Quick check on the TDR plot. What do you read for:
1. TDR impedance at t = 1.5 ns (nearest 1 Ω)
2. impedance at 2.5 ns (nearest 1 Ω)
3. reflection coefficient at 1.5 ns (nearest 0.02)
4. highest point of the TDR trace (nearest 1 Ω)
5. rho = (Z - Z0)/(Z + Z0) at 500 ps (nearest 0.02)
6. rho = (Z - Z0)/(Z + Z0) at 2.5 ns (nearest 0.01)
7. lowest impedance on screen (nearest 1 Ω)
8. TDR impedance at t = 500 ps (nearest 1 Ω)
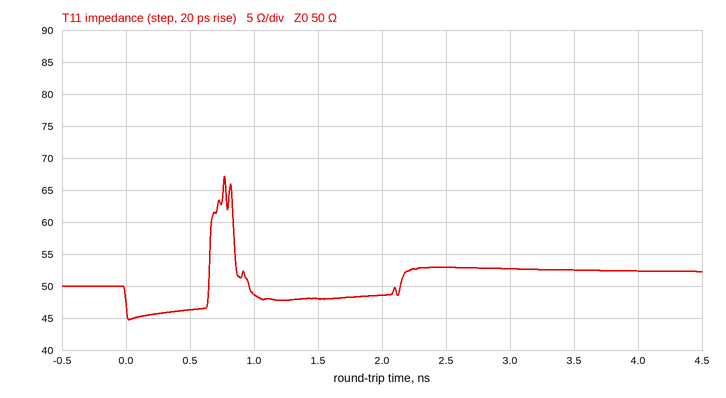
48 Ω
53 Ω
-0.02
67 Ω
-0.04
+0.03
45 Ω
46 Ω
